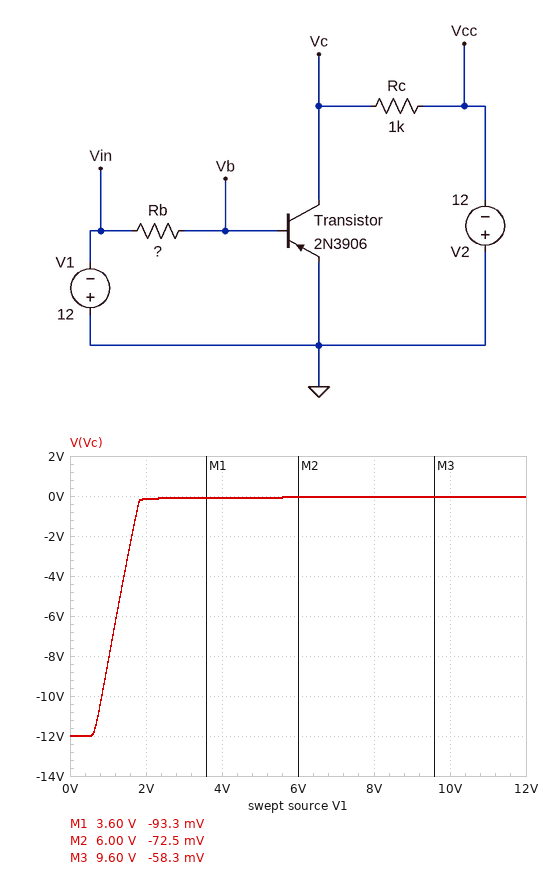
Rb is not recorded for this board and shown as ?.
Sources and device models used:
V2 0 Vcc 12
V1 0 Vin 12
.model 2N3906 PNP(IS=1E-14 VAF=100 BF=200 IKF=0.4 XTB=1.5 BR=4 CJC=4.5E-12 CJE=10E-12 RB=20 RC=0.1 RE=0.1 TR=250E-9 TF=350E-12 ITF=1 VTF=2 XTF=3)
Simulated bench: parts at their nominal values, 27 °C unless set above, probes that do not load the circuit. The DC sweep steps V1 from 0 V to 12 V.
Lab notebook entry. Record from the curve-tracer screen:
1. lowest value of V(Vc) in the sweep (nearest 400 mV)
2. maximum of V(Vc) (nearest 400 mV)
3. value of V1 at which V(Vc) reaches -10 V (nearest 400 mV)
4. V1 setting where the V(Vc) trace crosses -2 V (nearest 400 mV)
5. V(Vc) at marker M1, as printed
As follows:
-12.0 V
0 V
800 mV
1.6 V
-93.3 mV
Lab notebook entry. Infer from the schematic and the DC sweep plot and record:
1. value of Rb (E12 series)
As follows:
18 kΩ
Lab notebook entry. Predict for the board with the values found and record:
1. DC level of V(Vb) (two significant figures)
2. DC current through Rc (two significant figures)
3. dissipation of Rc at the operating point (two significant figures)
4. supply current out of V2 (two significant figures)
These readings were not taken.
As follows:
-740 mV
12 mA
140 mW
12 mA
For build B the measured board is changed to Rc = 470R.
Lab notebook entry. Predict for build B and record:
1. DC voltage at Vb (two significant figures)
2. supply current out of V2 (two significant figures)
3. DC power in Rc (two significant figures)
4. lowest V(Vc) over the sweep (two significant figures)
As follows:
-760 mV
25 mA
300 mW
-12 V
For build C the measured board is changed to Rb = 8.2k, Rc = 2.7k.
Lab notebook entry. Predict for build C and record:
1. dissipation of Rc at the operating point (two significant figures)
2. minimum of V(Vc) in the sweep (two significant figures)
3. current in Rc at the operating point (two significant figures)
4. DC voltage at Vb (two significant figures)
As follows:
53 mW
-12 V
4.4 mA
-750 mV
